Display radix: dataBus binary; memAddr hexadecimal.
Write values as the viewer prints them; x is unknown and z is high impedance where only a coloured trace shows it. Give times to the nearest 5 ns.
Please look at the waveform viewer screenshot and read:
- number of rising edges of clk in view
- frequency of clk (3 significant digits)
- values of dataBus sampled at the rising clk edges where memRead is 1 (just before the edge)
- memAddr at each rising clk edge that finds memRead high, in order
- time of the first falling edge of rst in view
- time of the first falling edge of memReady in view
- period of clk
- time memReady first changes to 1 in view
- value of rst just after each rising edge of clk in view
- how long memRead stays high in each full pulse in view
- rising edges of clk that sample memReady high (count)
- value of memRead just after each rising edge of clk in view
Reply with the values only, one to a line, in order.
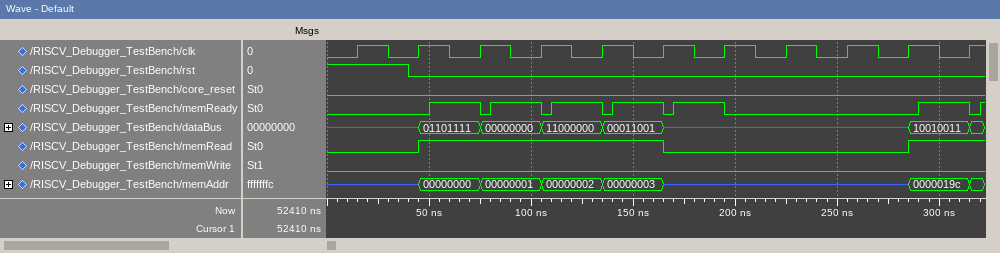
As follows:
11
33.3 MHz
01101111, 00000000, 11000000, 00011001, 10010011
00000000, 00000001, 00000002, 00000003, 0000019c
40 ns
75 ns
30 ns
50 ns
1 0 0 0 0 0 0 0 0 0 0
120 ns
6
0 1 1 1 1 0 0 0 0 1 1
